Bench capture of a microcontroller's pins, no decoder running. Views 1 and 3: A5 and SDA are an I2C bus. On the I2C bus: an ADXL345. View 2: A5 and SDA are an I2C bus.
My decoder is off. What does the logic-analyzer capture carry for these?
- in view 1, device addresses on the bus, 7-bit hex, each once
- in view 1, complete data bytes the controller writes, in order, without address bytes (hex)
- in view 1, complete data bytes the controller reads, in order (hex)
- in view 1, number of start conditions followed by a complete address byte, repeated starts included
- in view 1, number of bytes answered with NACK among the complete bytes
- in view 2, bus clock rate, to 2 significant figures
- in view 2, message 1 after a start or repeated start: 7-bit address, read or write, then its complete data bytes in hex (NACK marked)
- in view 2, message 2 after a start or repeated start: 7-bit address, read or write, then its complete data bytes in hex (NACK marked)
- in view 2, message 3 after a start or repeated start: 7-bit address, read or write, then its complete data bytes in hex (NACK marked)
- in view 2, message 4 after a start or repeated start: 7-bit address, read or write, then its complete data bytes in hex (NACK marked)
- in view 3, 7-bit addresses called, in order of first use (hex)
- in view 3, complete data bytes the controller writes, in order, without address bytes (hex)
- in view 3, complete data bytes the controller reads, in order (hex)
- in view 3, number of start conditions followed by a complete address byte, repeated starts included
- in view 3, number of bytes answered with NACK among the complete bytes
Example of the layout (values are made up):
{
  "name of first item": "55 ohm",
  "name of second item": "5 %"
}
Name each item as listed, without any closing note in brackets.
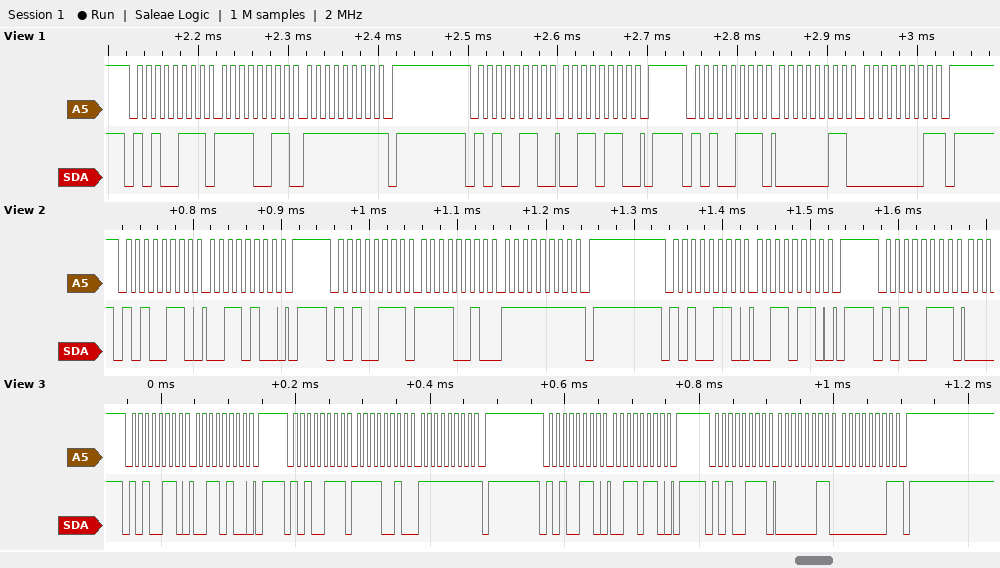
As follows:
{
  "in view 1, device addresses on the bus, 7-bit hex, each once": "0x53",
  "in view 1, complete data bytes the controller writes, in order, without address bytes": "36",
  "in view 1, complete data bytes the controller reads, in order": "F3 FF 03 01",
  "in view 1, number of start conditions followed by a complete address byte, repeated starts included": "3",
  "in view 1, number of bytes answered with NACK among the complete bytes": "2",
  "in view 2, bus clock rate, to 2 significant figures": "100 kHz",
  "in view 2, message 1 after a start or repeated start: 7-bit address, read or write, then its complete data bytes in hex": "0x53 write: 34",
  "in view 2, message 2 after a start or repeated start: 7-bit address, read or write, then its complete data bytes in hex": "0x53 read: F2 FF NACK",
  "in view 2, message 3 after a start or repeated start: 7-bit address, read or write, then its complete data bytes in hex": "0x53 write: 36",
  "in view 2, message 4 after a start or repeated start: 7-bit address, read or write, then its complete data bytes in hex": "0x53 read",
  "in view 3, 7-bit addresses called, in order of first use": "0x53",
  "in view 3, complete data bytes the controller writes, in order, without address bytes": "34 36",
  "in view 3, complete data bytes the controller reads, in order": "F2 FF 03 01",
  "in view 3, number of start conditions followed by a complete address byte, repeated starts included": "4",
  "in view 3, number of bytes answered with NACK among the complete bytes": "2"
}
